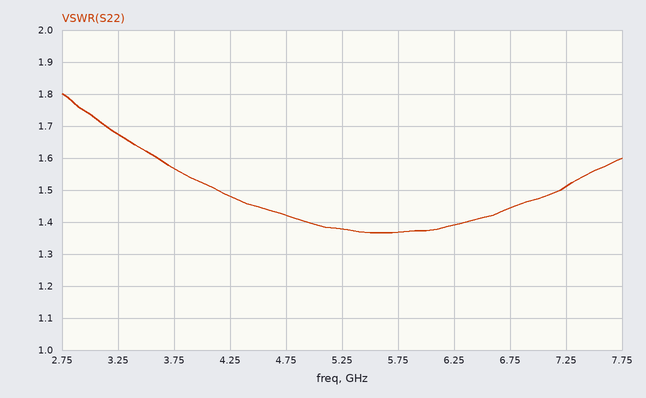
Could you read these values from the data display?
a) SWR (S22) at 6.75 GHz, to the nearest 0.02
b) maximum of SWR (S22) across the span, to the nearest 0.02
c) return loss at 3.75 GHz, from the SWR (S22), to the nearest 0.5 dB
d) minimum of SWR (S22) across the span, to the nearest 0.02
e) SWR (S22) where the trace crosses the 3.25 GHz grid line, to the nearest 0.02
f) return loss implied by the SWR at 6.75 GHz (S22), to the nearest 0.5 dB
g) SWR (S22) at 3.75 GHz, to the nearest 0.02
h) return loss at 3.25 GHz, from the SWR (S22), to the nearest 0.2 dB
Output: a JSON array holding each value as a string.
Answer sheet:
["1.44", "1.80", "13.0 dB", "1.36", "1.68", "15.0 dB", "1.56", "12.0 dB"]
